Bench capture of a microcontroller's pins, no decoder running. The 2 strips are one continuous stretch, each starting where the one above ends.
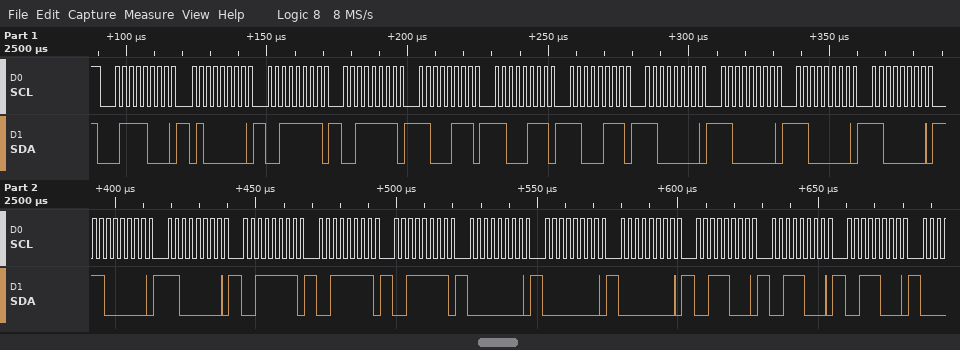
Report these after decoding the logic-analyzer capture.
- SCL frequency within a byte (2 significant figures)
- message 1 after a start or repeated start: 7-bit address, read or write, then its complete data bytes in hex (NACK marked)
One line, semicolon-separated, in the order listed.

400 kHz; 0x3C write: 40 3F 3F C7 C7 C7 C0 C0 C0 C0 C0 C0 3F 3F 3F 00 00 00 38 38 38
